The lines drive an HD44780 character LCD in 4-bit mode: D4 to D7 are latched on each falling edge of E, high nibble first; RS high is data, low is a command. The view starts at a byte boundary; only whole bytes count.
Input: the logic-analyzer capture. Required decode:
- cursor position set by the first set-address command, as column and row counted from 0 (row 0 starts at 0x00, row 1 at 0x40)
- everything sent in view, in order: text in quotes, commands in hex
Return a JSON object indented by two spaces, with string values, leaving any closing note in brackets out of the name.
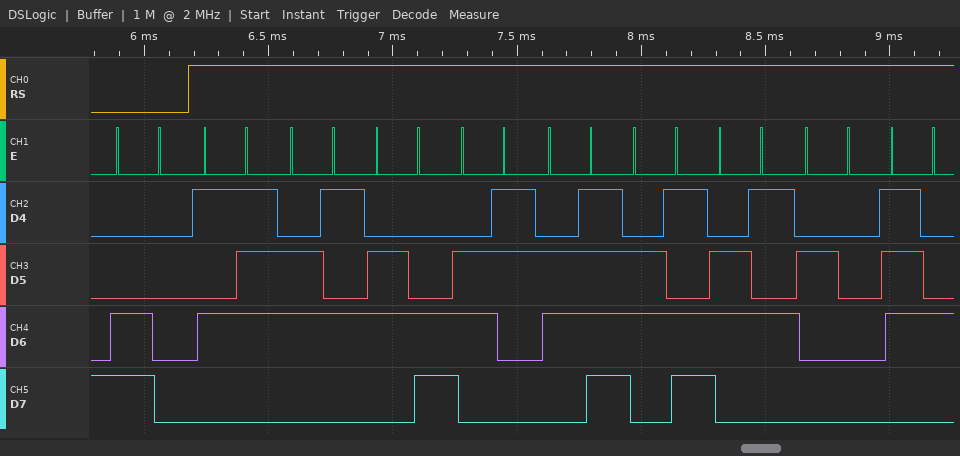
{
  "cursor position set by the first set-address command, as column and row counted from 0": "column 0, row 1",
  "everything sent in view, in order: text in quotes, commands in hex": "0xC0 \"Welcome t\""
}
